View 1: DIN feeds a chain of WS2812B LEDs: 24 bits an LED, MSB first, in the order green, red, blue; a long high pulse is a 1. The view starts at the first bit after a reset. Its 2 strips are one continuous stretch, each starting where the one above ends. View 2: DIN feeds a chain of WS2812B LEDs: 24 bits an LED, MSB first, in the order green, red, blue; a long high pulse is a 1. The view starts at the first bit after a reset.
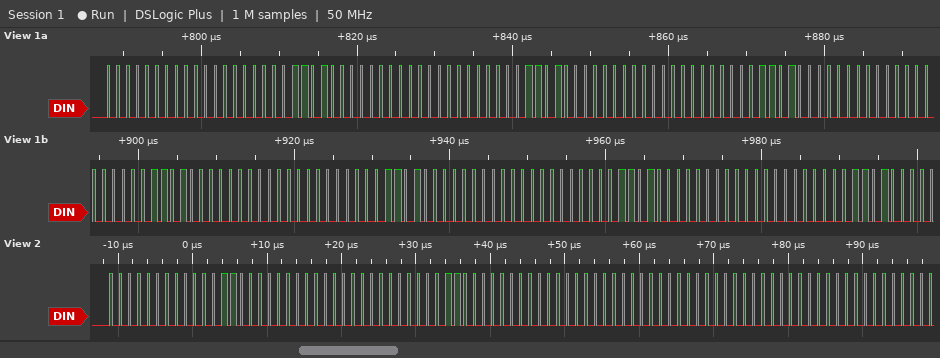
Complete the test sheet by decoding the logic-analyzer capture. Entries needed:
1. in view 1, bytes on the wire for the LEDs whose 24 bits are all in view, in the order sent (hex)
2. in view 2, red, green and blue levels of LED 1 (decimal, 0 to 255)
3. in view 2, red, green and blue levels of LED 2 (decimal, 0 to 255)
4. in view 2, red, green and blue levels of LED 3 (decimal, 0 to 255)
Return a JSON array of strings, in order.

["00 00 1A 00 00 1A 00 00 1A 00 00 1A 00 00 1A 00 00 1A 00 00 1A", "12, 0, 0", "12, 0, 0", "0, 0, 0"]
